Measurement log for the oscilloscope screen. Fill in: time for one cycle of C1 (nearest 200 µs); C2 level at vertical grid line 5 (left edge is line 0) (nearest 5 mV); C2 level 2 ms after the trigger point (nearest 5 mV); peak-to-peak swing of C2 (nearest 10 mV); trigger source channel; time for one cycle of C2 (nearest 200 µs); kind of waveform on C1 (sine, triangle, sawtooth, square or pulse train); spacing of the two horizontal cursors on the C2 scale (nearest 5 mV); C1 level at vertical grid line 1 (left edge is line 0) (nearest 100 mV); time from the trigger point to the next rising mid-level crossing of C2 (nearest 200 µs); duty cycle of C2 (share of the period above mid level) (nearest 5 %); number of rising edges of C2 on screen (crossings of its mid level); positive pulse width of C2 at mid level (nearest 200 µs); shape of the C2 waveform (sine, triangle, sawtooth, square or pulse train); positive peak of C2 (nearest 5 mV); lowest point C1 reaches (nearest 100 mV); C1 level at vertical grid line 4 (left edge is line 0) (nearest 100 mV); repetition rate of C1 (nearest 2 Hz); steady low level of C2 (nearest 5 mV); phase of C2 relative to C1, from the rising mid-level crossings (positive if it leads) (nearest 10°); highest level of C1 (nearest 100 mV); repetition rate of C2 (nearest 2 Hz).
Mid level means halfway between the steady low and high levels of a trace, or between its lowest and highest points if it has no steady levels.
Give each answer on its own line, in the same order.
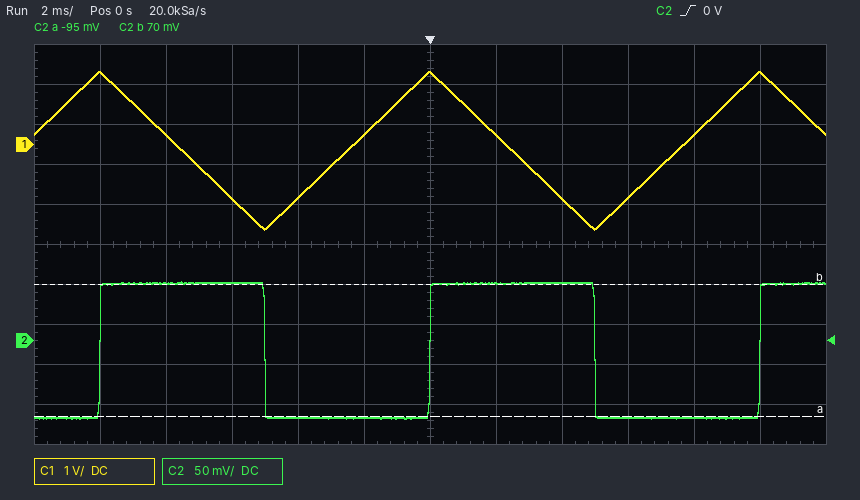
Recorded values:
10.0 ms
-95 mV
70 mV
170 mV
C2
10.0 ms
triangle
165 mV
1.8 V
10.0 ms
50 %
3
5.0 ms
square
75 mV
-2.1 V
-1.3 V
100 Hz
-95 mV
-90°
1.8 V
100 Hz
